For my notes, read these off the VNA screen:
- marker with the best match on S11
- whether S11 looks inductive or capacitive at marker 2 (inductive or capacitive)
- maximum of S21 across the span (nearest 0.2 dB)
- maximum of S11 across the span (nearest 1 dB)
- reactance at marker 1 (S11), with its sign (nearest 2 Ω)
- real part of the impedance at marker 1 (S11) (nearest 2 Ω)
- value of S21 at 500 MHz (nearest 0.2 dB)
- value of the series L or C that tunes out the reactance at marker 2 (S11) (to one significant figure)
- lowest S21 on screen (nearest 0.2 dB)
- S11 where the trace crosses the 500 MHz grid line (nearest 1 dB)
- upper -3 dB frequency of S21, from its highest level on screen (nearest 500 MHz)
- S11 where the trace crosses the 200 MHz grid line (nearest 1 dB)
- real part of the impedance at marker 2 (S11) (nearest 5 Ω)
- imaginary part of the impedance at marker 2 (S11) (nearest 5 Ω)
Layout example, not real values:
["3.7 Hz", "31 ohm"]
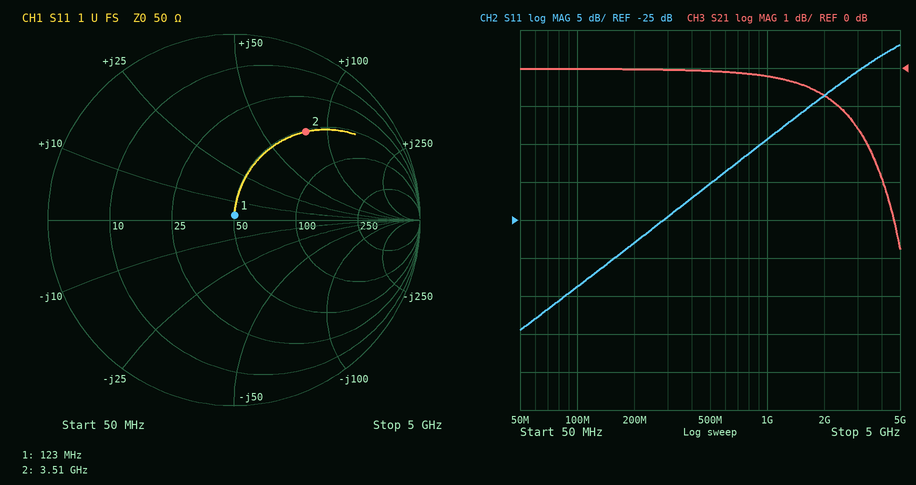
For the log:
["marker 1", "inductive", "0.0 dB", "-2 dB", "+2 Ω", "50 Ω", "0.0 dB", "600 fF", "-4.8 dB", "-20 dB", "4.0 GHz", "-28 dB", "50 Ω", "+80 Ω"]
